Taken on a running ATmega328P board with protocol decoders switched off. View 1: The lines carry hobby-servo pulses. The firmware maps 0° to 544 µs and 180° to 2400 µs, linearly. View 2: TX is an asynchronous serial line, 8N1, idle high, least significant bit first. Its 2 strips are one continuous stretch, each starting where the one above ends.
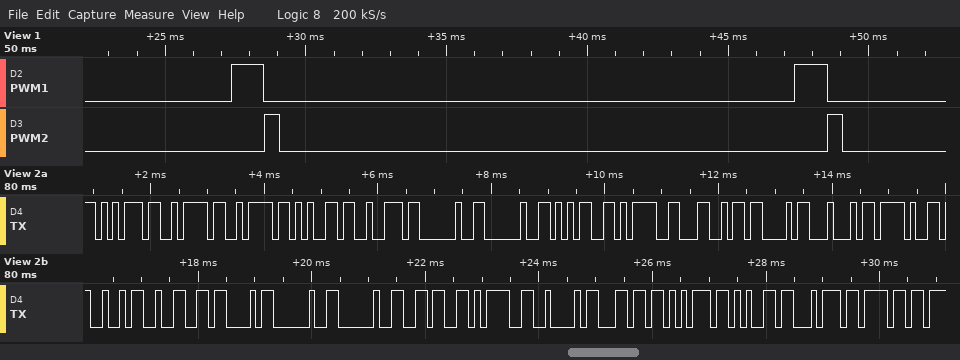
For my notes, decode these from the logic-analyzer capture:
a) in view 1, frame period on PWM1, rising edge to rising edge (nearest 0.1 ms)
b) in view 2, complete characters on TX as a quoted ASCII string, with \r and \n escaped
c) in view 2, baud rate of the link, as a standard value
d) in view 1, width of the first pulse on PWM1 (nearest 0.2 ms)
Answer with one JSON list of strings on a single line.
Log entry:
["20.0 ms", "\"uzzer  5=LCD/I2C  6=Blueto\"", "9600 baud", "1.2 ms"]
